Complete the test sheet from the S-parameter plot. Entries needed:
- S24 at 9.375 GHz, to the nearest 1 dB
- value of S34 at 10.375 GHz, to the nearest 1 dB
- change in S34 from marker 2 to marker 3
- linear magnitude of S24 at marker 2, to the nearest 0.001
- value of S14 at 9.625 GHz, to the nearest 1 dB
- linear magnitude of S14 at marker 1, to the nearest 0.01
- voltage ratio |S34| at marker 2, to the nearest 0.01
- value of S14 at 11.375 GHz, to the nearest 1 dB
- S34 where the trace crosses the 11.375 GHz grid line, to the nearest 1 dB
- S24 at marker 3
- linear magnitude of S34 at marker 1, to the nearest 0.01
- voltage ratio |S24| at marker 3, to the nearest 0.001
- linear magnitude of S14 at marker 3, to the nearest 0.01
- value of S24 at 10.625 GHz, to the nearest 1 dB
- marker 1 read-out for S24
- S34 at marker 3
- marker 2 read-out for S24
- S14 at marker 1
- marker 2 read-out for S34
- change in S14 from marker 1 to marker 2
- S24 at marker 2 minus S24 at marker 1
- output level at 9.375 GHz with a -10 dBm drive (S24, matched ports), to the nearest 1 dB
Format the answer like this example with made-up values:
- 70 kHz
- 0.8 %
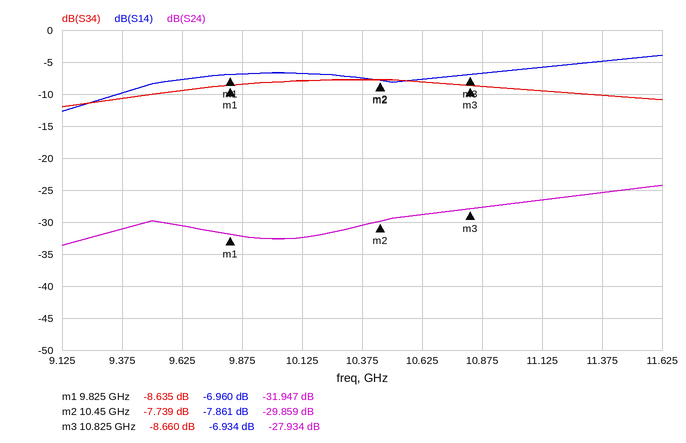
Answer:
- -31 dB
- -8 dB
- -0.921 dB
- 0.032
- -8 dB
- 0.45
- 0.41
- -5 dB
- -10 dB
- -27.934 dB
- 0.37
- 0.040
- 0.45
- -29 dB
- -31.947 dB
- -8.660 dB
- -29.859 dB
- -6.960 dB
- -7.739 dB
- -0.901 dB
- 2.088 dB
- -41 dBm
